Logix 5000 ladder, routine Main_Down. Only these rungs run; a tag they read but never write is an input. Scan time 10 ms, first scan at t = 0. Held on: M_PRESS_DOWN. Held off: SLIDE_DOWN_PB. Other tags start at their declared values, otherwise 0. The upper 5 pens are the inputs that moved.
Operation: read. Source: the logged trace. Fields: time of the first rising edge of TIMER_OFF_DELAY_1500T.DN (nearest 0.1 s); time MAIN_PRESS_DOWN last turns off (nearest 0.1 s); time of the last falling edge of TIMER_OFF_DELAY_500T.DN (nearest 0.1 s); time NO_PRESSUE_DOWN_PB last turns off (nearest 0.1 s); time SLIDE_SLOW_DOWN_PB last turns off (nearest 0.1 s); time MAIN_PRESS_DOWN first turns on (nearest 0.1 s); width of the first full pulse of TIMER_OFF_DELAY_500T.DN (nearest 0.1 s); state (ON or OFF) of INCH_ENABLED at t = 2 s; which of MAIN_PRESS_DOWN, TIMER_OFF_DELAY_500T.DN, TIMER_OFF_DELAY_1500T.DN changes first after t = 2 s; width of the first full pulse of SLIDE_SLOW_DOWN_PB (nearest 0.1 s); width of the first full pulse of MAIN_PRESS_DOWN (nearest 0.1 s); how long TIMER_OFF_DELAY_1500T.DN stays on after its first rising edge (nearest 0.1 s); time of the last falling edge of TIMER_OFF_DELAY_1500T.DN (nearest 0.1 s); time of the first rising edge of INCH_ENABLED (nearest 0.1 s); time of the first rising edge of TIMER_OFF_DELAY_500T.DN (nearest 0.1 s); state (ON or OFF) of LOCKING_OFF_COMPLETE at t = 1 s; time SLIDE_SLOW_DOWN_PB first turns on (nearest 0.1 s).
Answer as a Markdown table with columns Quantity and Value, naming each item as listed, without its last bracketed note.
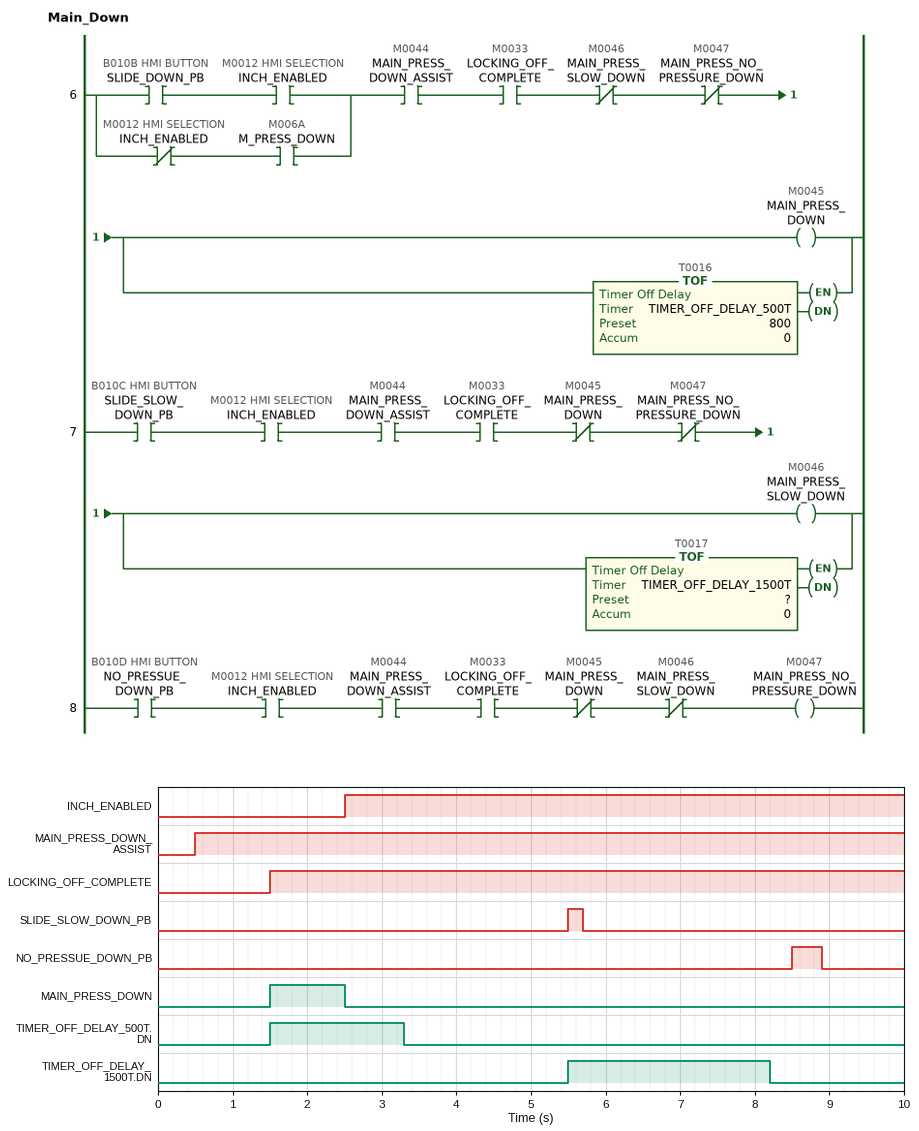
| Quantity | Value |
|---|---|
| time of the first rising edge of TIMER_OFF_DELAY_1500T.DN | 5.5 s |
| time MAIN_PRESS_DOWN last turns off | 2.5 s |
| time of the last falling edge of TIMER_OFF_DELAY_500T.DN | 3.3 s |
| time NO_PRESSUE_DOWN_PB last turns off | 8.9 s |
| time SLIDE_SLOW_DOWN_PB last turns off | 5.7 s |
| time MAIN_PRESS_DOWN first turns on | 1.5 s |
| width of the first full pulse of TIMER_OFF_DELAY_500T.DN | 1.8 s |
| state (ON or OFF) of INCH_ENABLED at t = 2 s | OFF |
| which of MAIN_PRESS_DOWN, TIMER_OFF_DELAY_500T.DN, TIMER_OFF_DELAY_1500T.DN changes first after t = 2 s | MAIN_PRESS_DOWN |
| width of the first full pulse of SLIDE_SLOW_DOWN_PB | 0.2 s |
| width of the first full pulse of MAIN_PRESS_DOWN | 1.0 s |
| how long TIMER_OFF_DELAY_1500T.DN stays on after its first rising edge | 2.7 s |
| time of the last falling edge of TIMER_OFF_DELAY_1500T.DN | 8.2 s |
| time of the first rising edge of INCH_ENABLED | 2.5 s |
| time of the first rising edge of TIMER_OFF_DELAY_500T.DN | 1.5 s |
| state (ON or OFF) of LOCKING_OFF_COMPLETE at t = 1 s | OFF |
| time SLIDE_SLOW_DOWN_PB first turns on | 5.5 s |
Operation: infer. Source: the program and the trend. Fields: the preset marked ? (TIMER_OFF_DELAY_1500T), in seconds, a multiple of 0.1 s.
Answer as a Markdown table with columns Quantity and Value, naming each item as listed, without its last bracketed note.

| Quantity | Value |
|---|---|
| the preset marked ? (TIMER_OFF_DELAY_1500T), in seconds, a multiple of 0.1 s | 2.5 s |
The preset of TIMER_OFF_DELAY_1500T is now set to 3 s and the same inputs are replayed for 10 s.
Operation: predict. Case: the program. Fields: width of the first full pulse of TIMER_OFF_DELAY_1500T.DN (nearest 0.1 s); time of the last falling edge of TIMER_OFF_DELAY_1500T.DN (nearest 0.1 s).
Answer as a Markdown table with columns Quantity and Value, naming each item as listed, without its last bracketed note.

| Quantity | Value |
|---|---|
| width of the first full pulse of TIMER_OFF_DELAY_1500T.DN | 3.2 s |
| time of the last falling edge of TIMER_OFF_DELAY_1500T.DN | 8.7 s |
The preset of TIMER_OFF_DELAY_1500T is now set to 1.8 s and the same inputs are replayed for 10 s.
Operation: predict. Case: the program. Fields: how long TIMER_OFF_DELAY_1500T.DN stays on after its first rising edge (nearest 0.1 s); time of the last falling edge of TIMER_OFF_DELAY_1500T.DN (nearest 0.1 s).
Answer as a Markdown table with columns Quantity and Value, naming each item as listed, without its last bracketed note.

| Quantity | Value |
|---|---|
| how long TIMER_OFF_DELAY_1500T.DN stays on after its first rising edge | 2.0 s |
| time of the last falling edge of TIMER_OFF_DELAY_1500T.DN | 7.5 s |
